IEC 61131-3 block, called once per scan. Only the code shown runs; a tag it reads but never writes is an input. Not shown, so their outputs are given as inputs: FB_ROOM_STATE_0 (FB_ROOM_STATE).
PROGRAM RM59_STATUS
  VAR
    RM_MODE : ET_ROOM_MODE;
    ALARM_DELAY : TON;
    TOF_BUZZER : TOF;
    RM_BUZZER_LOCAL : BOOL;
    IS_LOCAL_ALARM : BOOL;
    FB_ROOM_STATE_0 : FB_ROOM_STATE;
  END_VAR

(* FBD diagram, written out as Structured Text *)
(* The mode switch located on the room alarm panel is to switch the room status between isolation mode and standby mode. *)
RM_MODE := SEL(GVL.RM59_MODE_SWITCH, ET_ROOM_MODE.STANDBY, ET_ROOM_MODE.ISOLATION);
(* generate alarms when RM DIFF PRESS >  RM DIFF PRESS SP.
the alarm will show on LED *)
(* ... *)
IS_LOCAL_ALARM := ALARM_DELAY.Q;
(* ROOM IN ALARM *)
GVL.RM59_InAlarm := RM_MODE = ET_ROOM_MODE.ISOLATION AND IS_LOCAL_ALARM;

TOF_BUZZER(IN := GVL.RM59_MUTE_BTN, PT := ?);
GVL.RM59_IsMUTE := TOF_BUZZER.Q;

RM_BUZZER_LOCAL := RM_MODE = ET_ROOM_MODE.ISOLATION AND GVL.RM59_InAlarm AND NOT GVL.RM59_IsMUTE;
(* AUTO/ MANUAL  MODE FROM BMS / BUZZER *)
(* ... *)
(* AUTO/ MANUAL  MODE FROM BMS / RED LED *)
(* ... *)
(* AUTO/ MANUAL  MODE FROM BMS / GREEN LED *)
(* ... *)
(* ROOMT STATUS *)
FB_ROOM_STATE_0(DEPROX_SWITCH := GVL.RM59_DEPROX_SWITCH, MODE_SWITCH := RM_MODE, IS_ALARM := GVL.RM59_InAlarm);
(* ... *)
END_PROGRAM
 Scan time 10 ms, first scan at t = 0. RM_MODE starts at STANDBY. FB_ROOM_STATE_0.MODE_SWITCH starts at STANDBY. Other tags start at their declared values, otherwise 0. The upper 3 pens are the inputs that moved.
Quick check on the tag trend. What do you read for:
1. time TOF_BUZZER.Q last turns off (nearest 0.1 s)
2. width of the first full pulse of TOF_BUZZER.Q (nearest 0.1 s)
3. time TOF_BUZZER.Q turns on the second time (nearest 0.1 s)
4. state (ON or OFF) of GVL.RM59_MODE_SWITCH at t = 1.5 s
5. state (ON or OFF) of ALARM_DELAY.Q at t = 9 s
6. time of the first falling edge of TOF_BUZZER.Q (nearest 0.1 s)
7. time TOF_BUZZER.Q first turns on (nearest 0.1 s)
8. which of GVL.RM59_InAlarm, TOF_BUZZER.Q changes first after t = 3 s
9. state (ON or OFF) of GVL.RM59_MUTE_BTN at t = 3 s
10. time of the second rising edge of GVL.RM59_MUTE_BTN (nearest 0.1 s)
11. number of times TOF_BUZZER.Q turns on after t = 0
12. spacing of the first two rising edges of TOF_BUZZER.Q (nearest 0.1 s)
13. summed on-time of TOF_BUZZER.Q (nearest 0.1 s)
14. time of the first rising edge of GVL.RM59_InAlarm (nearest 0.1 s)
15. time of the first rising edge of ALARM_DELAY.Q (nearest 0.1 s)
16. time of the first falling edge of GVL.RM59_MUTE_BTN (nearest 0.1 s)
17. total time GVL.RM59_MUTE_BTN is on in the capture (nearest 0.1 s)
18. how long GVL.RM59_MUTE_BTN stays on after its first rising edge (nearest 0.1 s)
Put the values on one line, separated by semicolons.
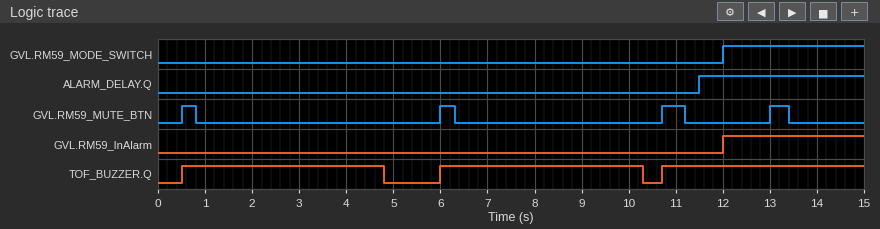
10.3 s; 4.3 s; 6.0 s; OFF; OFF; 4.8 s; 0.5 s; TOF_BUZZER.Q; OFF; 6.0 s; 3; 5.5 s; 12.9 s; 12.0 s; 11.5 s; 0.8 s; 1.5 s; 0.3 s
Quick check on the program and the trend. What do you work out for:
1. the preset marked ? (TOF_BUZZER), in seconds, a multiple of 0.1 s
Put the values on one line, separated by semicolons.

4.0 s
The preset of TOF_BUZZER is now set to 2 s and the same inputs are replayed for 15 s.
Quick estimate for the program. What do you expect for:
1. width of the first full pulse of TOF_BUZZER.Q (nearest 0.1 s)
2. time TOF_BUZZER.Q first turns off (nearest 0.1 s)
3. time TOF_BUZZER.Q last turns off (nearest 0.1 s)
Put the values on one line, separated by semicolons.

2.3 s; 2.8 s; 8.3 s
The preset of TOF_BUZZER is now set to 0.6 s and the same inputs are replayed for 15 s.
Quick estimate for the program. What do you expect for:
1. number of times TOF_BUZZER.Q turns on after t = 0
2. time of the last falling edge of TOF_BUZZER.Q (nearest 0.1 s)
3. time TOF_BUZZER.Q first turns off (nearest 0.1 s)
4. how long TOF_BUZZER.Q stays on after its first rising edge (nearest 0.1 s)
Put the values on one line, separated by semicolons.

4; 14.0 s; 1.4 s; 0.9 s
